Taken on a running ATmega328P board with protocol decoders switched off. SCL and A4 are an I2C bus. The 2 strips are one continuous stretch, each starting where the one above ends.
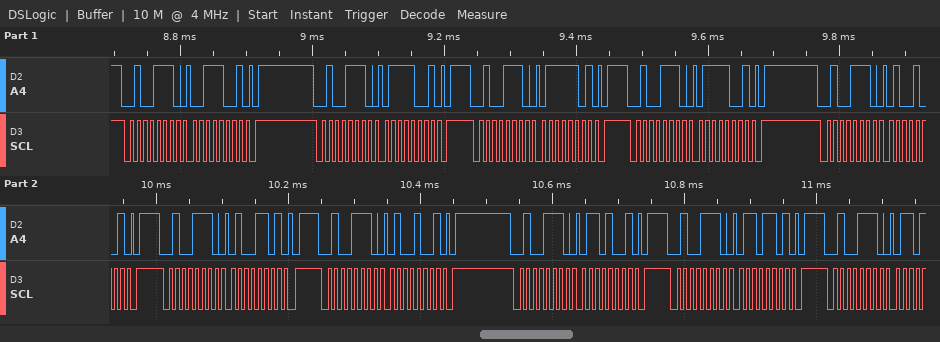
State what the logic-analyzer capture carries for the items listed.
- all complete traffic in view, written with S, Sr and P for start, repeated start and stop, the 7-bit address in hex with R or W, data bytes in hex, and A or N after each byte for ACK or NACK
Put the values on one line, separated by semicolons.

S 27W A 39 A P S 27W A 79 A P S 27W A 7D A P S 27W A 79 A P S 27W A 49 A P S 27W A 4D A P S 27W A 49 A P S 27W A 69 A P S 27W A 6D A P S 27W A
